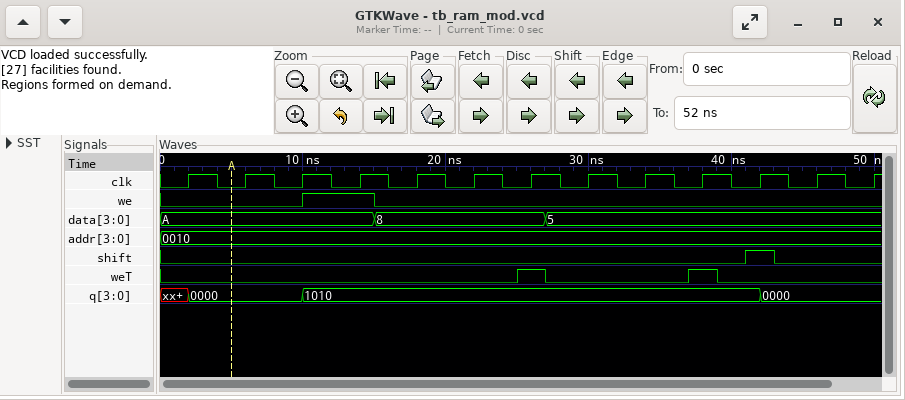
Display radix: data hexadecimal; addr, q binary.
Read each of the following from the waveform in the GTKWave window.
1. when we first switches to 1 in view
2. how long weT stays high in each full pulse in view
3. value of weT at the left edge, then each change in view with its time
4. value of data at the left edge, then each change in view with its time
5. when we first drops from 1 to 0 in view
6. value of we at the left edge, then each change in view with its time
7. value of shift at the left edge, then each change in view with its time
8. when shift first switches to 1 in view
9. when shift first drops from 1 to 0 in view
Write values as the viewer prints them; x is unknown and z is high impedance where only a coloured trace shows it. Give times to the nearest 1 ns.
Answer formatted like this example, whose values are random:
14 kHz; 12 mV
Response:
10 ns; 2 ns, 2 ns; 0, 1 at 25 ns, 0 at 27 ns, 1 at 37 ns, 0 at 39 ns; A, 8 at 15 ns, 5 at 27 ns; 15 ns; 0, 1 at 10 ns, 0 at 15 ns; 0, 1 at 41 ns, 0 at 43 ns; 41 ns; 43 ns
